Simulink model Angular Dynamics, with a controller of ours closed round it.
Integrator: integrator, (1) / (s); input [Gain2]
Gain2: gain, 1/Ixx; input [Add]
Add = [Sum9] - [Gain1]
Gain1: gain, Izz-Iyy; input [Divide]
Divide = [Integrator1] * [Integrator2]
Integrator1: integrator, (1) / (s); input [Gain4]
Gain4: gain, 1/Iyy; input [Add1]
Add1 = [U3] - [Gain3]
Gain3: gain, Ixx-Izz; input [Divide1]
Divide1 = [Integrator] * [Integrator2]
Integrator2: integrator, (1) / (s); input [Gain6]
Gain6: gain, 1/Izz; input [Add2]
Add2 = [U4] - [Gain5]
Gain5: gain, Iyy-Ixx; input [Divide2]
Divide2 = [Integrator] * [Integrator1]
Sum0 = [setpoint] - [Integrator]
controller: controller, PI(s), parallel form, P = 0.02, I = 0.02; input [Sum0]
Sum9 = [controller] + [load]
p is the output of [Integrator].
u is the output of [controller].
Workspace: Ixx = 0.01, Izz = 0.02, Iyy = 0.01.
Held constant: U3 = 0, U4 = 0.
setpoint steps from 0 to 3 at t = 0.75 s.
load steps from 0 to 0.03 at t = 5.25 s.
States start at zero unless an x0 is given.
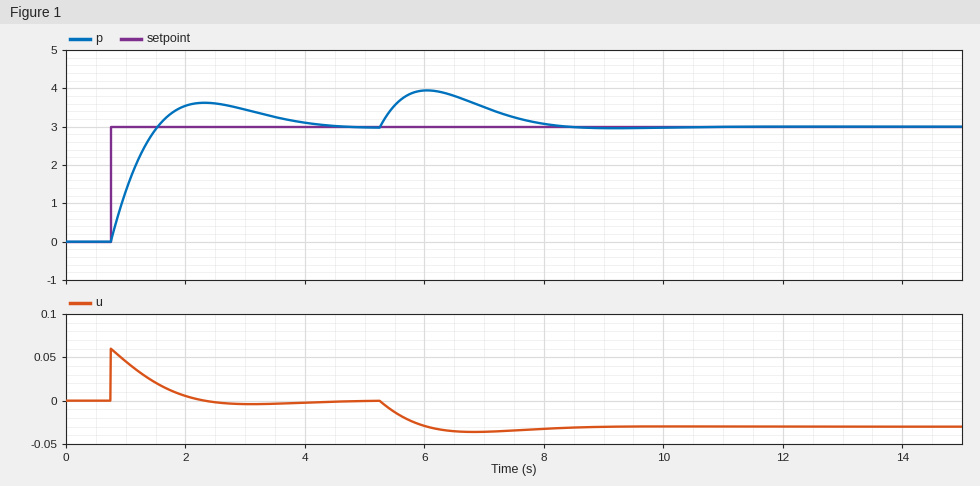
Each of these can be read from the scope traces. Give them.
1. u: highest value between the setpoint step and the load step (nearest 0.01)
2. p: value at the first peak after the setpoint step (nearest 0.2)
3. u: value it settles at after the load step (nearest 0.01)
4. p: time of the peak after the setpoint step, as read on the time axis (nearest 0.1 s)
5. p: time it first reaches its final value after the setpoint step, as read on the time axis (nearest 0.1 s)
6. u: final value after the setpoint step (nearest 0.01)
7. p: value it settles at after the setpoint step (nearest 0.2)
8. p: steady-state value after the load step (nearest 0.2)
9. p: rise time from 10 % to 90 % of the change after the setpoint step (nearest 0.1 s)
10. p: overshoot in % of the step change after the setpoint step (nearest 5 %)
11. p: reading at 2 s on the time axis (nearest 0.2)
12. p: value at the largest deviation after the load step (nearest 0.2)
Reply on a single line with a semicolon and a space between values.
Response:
0.06; 3.6; -0.03; 2.3 s; 1.5 s; 0.00; 3.0; 3.0; 0.6 s; 20 %; 3.6; 4.0
